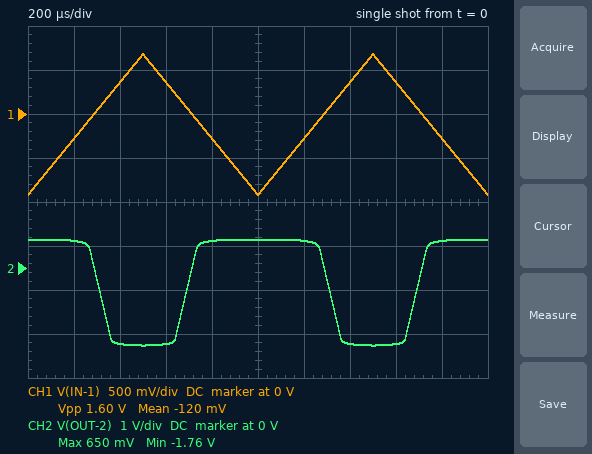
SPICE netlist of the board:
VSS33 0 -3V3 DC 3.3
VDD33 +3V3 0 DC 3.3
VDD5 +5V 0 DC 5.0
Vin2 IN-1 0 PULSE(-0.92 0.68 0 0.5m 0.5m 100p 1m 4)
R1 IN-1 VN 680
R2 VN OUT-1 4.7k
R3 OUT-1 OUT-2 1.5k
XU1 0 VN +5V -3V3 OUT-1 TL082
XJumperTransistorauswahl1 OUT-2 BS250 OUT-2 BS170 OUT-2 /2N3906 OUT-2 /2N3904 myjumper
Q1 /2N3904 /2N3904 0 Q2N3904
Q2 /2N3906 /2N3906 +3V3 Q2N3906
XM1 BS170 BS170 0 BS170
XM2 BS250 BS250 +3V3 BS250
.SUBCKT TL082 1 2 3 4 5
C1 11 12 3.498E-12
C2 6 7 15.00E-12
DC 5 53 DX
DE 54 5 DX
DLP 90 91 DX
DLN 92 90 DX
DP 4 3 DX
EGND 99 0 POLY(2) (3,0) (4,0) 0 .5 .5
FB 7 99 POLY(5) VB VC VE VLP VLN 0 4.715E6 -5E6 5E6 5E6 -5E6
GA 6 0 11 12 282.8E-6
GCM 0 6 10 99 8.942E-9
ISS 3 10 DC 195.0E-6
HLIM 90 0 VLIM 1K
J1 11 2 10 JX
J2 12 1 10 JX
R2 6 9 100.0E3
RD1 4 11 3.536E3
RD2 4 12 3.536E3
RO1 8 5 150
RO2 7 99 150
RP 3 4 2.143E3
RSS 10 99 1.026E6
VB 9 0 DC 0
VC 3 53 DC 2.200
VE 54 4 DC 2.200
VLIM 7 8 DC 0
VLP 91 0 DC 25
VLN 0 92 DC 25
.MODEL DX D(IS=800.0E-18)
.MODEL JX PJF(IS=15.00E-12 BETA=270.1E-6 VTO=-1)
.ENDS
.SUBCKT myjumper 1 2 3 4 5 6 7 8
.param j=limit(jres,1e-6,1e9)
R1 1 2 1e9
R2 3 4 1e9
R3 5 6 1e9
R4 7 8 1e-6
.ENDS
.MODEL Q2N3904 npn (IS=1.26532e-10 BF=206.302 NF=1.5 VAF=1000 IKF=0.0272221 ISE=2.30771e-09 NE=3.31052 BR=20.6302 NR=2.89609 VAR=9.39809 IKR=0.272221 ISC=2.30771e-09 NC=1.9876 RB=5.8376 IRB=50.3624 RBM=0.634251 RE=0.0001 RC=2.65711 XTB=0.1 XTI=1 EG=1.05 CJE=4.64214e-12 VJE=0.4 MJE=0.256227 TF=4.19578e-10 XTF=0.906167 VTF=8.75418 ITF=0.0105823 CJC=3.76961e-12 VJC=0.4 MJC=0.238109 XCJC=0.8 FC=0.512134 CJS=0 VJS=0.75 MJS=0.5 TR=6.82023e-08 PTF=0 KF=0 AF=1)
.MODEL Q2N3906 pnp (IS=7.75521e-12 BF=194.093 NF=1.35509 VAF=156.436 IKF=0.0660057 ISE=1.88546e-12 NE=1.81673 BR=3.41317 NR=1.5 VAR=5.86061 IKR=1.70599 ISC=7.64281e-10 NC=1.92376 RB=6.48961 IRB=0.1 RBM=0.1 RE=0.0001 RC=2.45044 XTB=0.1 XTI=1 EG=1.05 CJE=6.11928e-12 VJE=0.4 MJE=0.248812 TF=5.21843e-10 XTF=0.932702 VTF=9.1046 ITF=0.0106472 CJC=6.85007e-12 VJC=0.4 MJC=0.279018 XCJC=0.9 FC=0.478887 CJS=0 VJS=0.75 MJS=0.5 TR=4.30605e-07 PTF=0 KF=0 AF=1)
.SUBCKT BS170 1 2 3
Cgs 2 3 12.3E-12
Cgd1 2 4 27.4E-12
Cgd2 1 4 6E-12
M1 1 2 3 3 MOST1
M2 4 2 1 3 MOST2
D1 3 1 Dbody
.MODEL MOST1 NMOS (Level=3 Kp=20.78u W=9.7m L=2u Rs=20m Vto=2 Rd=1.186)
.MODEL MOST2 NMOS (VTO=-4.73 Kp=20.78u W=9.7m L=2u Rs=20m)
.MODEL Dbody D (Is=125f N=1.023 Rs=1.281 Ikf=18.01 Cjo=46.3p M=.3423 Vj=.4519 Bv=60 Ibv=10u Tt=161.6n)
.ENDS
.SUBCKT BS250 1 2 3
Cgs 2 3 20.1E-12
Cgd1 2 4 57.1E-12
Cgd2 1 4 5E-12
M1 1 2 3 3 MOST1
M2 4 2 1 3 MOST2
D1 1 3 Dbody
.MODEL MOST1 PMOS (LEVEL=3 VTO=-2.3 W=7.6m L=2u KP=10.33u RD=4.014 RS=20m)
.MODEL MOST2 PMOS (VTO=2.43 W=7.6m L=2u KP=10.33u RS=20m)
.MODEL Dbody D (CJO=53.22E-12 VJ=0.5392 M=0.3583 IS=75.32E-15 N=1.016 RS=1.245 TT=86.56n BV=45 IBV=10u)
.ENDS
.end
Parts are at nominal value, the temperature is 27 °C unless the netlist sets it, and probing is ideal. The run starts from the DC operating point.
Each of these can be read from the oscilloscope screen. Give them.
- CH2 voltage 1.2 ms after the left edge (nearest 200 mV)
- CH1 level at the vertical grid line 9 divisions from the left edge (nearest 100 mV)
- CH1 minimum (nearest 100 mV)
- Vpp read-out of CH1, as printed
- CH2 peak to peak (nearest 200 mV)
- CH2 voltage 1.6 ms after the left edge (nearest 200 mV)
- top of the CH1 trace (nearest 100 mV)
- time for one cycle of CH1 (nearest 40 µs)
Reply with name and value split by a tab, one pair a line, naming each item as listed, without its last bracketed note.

CH2 voltage 1.2 ms after the left edge	600 mV
CH1 level at the vertical grid line 9 divisions from the left edge	-300 mV
CH1 minimum	-900 mV
Vpp read-out of CH1, as printed	1.60 V
CH2 peak to peak	2.4 V
CH2 voltage 1.6 ms after the left edge	-1.8 V
top of the CH1 trace	700 mV
time for one cycle of CH1	1.00 ms
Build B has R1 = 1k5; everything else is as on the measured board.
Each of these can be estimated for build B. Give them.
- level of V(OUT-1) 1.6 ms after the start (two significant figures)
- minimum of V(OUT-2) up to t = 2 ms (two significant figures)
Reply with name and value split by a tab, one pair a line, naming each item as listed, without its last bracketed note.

level of V(OUT-1) 1.6 ms after the start	-1.1 V
minimum of V(OUT-2) up to t = 2 ms	-1.7 V
